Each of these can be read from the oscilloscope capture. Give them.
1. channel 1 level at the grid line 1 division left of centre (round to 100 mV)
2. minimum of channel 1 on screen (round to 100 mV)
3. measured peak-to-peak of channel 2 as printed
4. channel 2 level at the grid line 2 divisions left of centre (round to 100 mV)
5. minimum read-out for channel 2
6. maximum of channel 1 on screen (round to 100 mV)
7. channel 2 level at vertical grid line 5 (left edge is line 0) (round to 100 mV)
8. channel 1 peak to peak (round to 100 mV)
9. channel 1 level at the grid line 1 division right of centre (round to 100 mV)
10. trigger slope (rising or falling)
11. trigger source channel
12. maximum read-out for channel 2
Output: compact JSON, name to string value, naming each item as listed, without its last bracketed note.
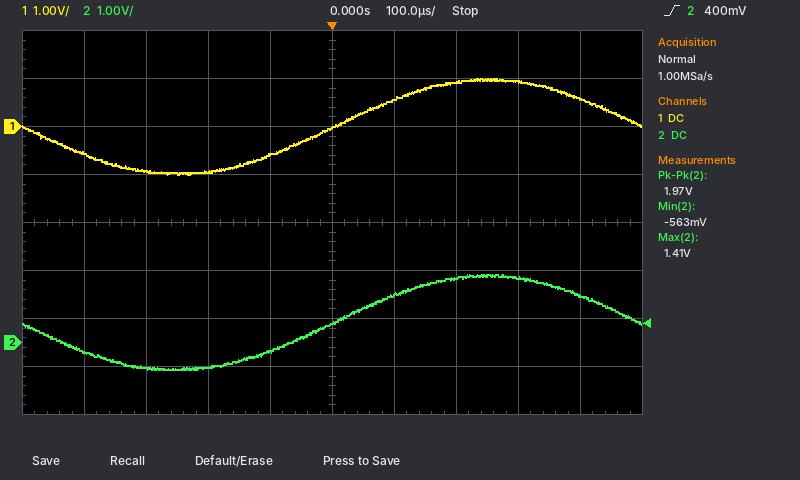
{"channel 1 level at the grid line 1 division left of centre": "-600 mV", "minimum of channel 1 on screen": "-1.0 V", "measured peak-to-peak of channel 2 as printed": "1.97 V", "channel 2 level at the grid line 2 divisions left of centre": "-500 mV", "minimum read-out for channel 2": "-563 mV", "maximum of channel 1 on screen": "1.0 V", "channel 2 level at vertical grid line 5 (left edge is line 0)": "400 mV", "channel 1 peak to peak": "2.0 V", "channel 1 level at the grid line 1 division right of centre": "600 mV", "trigger slope": "rising", "trigger source channel": "channel 2", "maximum read-out for channel 2": "1.41 V"}
